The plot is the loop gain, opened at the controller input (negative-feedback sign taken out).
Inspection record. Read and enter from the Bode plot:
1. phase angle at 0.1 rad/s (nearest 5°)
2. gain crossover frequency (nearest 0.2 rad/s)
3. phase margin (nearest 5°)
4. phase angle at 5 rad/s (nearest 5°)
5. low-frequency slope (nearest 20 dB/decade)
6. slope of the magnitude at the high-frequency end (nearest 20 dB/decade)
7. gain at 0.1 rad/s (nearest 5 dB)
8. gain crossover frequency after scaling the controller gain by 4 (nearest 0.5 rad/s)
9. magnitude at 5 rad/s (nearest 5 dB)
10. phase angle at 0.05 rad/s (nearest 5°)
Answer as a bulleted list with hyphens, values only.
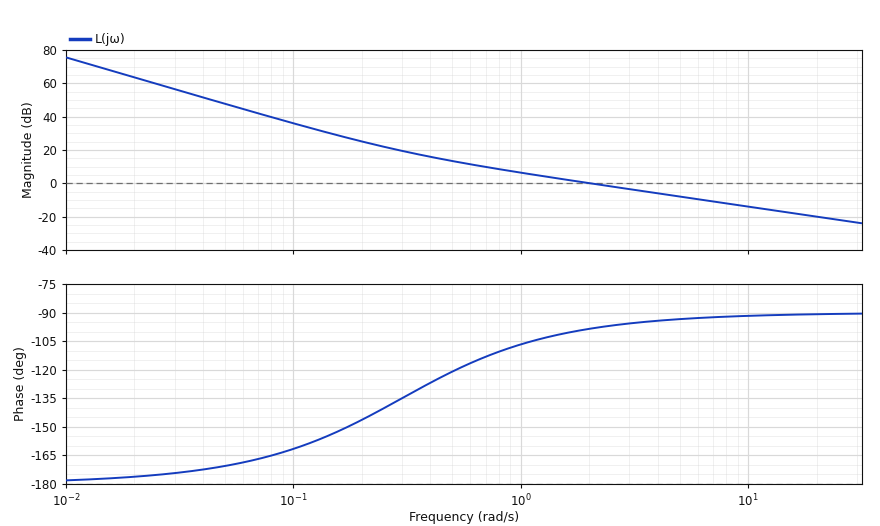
- -160°
- 2.0 rad/s
- 80°
- -95°
- -40 dB/decade
- -20 dB/decade
- 35 dB
- 8.0 rad/s
- -10 dB
- -170°
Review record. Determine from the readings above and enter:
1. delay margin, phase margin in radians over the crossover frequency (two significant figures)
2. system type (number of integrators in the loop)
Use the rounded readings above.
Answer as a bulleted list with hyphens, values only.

- 0.70 s
- 2
